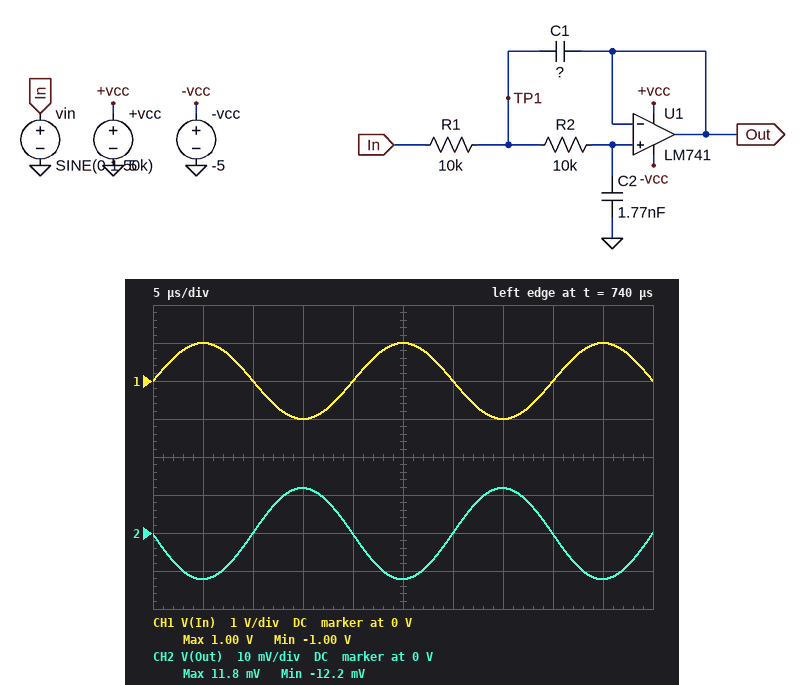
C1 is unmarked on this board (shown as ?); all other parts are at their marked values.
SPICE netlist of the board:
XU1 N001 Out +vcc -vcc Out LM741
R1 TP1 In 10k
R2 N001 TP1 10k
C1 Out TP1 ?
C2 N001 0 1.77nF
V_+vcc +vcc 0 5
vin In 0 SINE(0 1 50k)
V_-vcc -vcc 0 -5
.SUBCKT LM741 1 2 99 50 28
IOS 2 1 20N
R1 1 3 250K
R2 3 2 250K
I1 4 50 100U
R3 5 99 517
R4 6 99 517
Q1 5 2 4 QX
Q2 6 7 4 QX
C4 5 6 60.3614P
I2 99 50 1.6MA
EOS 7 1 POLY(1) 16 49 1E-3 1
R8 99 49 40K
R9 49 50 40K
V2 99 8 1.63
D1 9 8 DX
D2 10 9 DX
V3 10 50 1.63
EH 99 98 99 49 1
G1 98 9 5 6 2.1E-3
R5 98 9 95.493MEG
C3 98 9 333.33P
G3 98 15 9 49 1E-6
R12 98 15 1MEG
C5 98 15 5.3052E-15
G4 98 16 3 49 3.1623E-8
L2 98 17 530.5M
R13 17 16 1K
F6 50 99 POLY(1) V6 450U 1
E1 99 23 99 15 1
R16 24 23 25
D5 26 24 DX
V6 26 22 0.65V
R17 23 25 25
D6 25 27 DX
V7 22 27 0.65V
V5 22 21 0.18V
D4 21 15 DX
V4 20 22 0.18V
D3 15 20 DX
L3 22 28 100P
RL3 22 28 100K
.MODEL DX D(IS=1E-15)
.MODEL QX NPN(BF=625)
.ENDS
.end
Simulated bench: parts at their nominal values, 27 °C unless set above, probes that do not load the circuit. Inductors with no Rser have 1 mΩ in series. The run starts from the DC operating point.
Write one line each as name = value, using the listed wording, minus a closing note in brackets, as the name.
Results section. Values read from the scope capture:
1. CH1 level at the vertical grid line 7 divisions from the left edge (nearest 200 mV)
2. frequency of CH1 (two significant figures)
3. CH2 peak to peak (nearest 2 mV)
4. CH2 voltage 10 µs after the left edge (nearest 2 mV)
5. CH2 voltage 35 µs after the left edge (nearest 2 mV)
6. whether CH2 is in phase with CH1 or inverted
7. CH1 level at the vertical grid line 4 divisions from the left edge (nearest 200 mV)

CH1 level at the vertical grid line 7 divisions from the left edge = -1.0 V
frequency of CH1 = 50 kHz
CH2 peak to peak = 24 mV
CH2 voltage 10 µs after the left edge = 0 V
CH2 voltage 35 µs after the left edge = 12 mV
whether CH2 is in phase with CH1 or inverted = inverted
CH1 level at the vertical grid line 4 divisions from the left edge = 0 V
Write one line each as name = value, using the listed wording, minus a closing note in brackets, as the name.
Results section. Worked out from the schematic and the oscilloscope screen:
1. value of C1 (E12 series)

value of C1 = 4.7 nF
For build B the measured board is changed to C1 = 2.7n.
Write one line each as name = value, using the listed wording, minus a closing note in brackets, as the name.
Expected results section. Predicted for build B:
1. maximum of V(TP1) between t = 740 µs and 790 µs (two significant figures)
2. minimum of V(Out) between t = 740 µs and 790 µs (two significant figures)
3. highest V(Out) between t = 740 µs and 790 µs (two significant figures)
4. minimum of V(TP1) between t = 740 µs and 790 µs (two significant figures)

maximum of V(TP1) between t = 740 µs and 790 µs = 120 mV
minimum of V(Out) between t = 740 µs and 790 µs = -21 mV
highest V(Out) between t = 740 µs and 790 µs = 21 mV
minimum of V(TP1) between t = 740 µs and 790 µs = -120 mV
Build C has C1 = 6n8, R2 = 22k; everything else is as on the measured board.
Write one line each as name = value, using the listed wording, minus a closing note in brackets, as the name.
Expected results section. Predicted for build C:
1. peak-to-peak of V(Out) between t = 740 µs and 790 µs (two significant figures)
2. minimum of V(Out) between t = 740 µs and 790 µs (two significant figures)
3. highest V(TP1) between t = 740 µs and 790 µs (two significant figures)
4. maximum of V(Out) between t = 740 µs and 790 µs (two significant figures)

peak-to-peak of V(Out) between t = 740 µs and 790 µs = 7.7 mV
minimum of V(Out) between t = 740 µs and 790 µs = -4.7 mV
highest V(TP1) between t = 740 µs and 790 µs = 45 mV
maximum of V(Out) between t = 740 µs and 790 µs = 3.0 mV
